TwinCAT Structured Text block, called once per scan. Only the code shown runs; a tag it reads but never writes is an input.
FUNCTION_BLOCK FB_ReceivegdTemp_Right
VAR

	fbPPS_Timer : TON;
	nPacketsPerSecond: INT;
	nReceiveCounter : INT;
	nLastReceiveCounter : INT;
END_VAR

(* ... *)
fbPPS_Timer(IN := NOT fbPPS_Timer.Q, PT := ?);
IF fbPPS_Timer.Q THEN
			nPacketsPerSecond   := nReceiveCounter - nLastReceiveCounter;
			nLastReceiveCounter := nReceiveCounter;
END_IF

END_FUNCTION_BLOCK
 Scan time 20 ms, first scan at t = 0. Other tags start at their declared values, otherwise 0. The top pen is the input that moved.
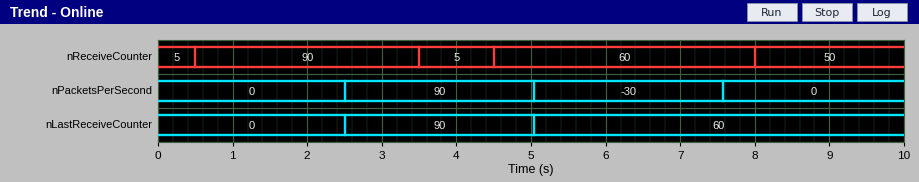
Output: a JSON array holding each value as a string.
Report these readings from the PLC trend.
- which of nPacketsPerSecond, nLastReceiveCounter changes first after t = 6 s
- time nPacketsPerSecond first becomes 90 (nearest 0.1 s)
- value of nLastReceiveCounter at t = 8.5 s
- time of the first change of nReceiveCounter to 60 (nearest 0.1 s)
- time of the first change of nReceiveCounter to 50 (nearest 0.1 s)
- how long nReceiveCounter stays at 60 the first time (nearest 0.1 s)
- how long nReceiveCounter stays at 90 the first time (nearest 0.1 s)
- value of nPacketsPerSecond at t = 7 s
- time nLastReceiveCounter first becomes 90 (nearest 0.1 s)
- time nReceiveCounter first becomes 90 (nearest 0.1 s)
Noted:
["nPacketsPerSecond", "2.5 s", "60", "4.5 s", "8.0 s", "3.5 s", "3.0 s", "-30", "2.5 s", "0.5 s"]
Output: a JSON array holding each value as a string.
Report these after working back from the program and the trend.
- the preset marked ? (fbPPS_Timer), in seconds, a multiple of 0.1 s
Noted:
["2.5 s"]
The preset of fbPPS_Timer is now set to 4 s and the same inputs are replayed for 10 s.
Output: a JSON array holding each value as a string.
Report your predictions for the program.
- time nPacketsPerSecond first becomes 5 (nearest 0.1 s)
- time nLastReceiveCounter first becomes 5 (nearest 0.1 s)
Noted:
["4.0 s", "4.0 s"]
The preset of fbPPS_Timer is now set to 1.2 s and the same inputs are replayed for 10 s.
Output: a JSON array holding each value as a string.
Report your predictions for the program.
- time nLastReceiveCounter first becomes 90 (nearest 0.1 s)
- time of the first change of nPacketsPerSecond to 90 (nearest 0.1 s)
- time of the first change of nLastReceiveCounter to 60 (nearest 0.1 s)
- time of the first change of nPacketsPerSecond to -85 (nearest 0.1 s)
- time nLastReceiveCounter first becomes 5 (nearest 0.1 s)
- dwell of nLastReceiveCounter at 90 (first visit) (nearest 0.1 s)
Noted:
["1.2 s", "1.2 s", "4.9 s", "3.7 s", "3.7 s", "2.5 s"]
